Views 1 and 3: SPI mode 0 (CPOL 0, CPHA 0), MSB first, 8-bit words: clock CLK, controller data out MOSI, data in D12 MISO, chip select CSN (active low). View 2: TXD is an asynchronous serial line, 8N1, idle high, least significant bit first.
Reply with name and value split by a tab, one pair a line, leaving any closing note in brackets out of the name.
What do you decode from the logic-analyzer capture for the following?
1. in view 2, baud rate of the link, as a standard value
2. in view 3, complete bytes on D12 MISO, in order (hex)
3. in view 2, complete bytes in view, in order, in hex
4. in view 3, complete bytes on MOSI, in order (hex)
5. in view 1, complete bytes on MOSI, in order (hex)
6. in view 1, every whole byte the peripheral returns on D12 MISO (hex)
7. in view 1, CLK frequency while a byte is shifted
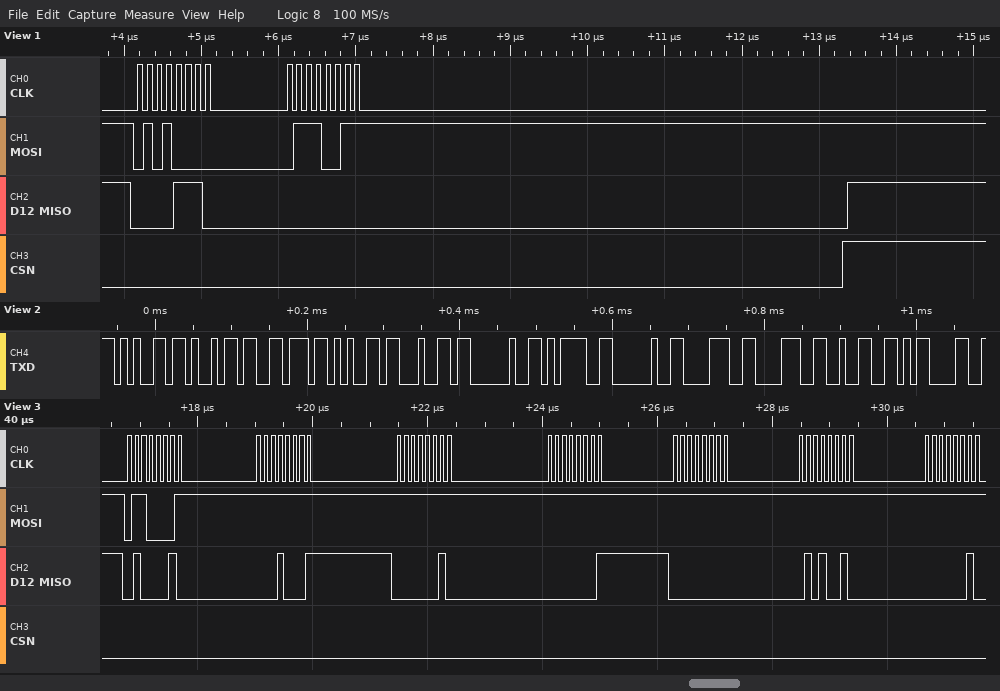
in view 2, baud rate of the link, as a standard value	115200 baud
in view 3, complete bytes on D12 MISO, in order	42 11 02 01 00 52 02
in view 2, complete bytes in view, in order, in hex	0x65 0x69 0x76 0x65 0x64 0x20 0x3D 0x20 0x38 0x38 0x32 0x0D
in view 3, complete bytes on MOSI, in order	61 FF FF FF FF FF FF
in view 1, complete bytes on MOSI, in order	0x50 0x73
in view 1, every whole byte the peripheral returns on D12 MISO	0x0E 0x00
in view 1, CLK frequency while a byte is shifted	8 MHz
